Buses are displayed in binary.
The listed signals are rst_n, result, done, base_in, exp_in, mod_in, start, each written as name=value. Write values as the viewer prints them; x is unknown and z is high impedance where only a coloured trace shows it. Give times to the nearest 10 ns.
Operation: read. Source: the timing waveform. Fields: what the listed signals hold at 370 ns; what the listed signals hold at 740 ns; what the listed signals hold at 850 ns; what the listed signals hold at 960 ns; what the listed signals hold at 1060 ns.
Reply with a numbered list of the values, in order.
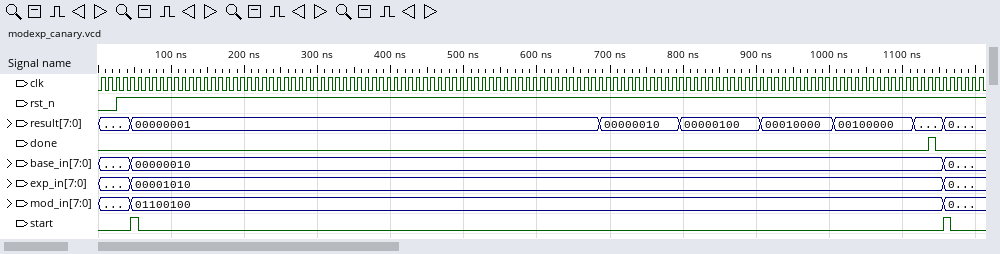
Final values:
1. rst_n=1, result=00000001, done=0, base_in=00000010, exp_in=00001010, mod_in=01100100, start=0
2. rst_n=1, result=00000010, done=0, base_in=00000010, exp_in=00001010, mod_in=01100100, start=0
3. rst_n=1, result=00000100, done=0, base_in=00000010, exp_in=00001010, mod_in=01100100, start=0
4. rst_n=1, result=00010000, done=0, base_in=00000010, exp_in=00001010, mod_in=01100100, start=0
5. rst_n=1, result=00100000, done=0, base_in=00000010, exp_in=00001010, mod_in=01100100, start=0
